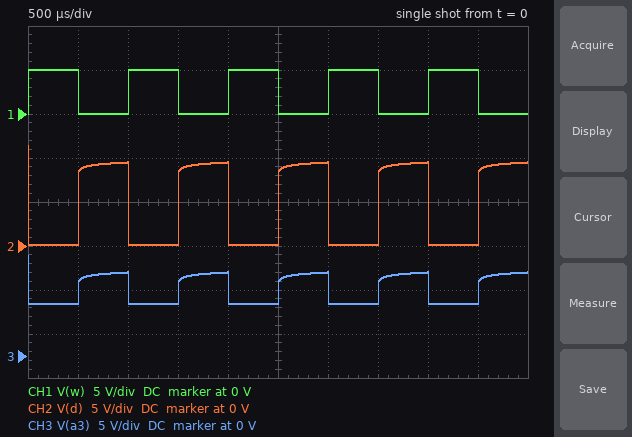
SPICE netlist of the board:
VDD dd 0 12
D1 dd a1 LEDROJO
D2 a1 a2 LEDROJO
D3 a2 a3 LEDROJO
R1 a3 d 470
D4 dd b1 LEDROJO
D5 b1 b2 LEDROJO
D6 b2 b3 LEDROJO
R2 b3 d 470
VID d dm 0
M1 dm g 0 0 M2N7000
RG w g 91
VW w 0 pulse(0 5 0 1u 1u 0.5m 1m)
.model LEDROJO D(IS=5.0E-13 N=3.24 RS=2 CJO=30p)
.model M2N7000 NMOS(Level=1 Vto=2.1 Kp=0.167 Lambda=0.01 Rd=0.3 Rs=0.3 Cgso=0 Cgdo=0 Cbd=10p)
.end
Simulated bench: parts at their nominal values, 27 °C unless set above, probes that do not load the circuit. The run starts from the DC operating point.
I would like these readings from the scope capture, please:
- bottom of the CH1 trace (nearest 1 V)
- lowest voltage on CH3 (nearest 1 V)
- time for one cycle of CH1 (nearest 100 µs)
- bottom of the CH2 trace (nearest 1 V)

0 V
6 V
1.0 ms
0 V
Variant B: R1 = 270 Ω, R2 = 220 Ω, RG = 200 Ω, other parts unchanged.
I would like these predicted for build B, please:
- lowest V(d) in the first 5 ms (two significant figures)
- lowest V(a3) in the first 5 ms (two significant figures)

120 mV
5.7 V
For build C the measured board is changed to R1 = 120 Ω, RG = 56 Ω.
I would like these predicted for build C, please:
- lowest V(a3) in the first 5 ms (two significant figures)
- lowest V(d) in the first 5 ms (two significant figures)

5.4 V
150 mV
